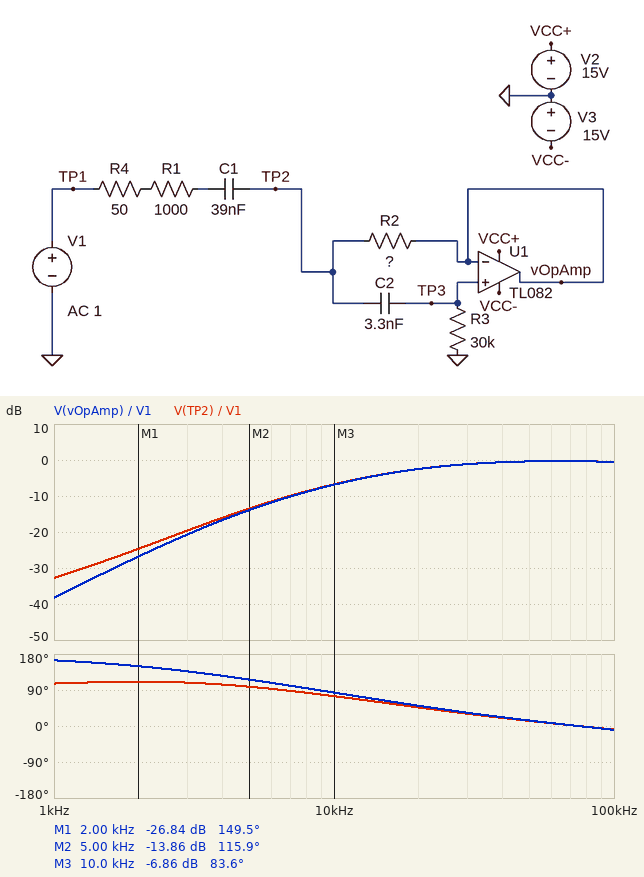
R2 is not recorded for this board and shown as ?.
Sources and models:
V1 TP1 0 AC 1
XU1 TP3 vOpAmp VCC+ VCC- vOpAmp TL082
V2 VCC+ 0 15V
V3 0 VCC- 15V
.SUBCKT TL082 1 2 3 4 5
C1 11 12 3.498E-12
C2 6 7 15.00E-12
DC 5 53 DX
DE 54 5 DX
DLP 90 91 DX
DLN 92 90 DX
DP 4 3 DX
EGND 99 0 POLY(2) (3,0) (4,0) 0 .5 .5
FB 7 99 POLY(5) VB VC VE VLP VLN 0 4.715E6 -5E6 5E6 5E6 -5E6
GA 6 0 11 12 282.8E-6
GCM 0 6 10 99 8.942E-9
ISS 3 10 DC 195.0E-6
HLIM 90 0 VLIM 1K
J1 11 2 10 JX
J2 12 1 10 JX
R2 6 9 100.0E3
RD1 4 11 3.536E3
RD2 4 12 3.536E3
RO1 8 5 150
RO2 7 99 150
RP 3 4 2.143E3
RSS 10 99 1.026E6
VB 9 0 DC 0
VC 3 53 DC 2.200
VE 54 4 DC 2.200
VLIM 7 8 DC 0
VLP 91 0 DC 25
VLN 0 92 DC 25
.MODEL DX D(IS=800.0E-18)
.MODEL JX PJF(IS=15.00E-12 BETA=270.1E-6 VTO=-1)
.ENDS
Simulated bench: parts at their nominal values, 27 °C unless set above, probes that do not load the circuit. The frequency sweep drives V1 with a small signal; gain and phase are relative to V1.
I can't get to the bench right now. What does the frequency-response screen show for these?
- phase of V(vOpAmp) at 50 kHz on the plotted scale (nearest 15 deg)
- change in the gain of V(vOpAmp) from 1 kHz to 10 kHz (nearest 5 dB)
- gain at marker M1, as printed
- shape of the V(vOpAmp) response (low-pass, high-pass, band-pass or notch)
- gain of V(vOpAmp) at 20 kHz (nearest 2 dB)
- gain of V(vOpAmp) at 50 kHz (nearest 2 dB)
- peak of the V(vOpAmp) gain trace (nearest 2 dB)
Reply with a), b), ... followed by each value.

a) 15 deg
b) 30 dB
c) -26.84 dB
d) high-pass
e) -2 dB
f) 0 dB
g) 0 dB
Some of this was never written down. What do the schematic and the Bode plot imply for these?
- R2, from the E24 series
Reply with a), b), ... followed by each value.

a) 82 Ω
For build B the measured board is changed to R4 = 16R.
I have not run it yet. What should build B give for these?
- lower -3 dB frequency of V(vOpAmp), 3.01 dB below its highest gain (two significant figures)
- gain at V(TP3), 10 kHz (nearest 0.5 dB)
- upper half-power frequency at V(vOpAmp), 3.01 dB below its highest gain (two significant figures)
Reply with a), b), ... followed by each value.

a) 16 kHz
b) -6.5 dB
c) 260 kHz
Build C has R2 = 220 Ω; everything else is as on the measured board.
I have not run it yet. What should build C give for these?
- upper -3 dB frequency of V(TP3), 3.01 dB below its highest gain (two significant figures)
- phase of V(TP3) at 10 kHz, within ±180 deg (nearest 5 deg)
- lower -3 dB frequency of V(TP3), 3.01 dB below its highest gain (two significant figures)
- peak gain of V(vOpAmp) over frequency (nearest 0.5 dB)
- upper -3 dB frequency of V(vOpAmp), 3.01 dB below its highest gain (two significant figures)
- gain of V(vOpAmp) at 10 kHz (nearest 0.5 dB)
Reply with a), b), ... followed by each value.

a) 620 kHz
b) 50 deg
c) 6.6 kHz
d) -0.5 dB
e) 600 kHz
f) -1.5 dB
